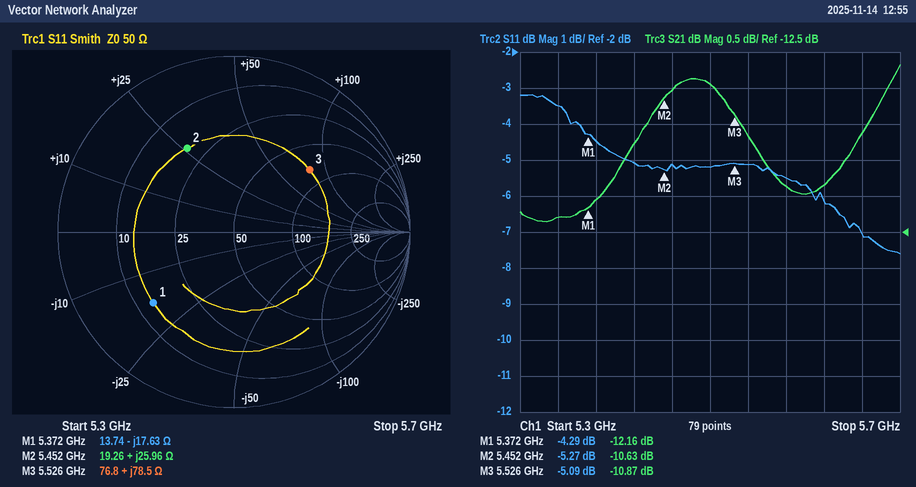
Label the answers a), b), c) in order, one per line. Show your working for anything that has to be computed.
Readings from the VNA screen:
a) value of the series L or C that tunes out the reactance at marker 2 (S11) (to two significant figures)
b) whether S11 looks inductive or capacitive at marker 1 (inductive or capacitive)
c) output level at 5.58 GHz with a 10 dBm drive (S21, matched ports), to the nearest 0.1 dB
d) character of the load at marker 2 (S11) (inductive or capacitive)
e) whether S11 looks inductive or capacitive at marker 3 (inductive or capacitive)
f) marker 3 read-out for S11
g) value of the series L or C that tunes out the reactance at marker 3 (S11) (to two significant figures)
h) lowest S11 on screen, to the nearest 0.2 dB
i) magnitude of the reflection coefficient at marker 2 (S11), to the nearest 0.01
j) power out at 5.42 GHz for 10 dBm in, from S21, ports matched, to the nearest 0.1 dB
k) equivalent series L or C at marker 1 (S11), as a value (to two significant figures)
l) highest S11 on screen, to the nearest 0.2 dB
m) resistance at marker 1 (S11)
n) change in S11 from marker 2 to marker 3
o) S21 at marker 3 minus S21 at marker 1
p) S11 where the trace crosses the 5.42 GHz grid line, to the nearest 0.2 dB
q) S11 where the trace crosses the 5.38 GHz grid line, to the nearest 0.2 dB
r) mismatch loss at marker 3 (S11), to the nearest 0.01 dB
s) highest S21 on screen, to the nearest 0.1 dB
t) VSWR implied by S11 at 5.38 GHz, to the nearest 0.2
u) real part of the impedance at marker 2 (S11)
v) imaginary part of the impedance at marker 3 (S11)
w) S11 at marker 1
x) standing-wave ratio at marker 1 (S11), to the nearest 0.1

a) C = 1/(2π × 5.452 GHz × 25.96 Ω) ≈ 1.1 pF
b) capacitive
c) 10 dBm + (-11.9 dB) = -1.9 dBm
d) inductive
e) inductive
f) -5.09 dB
g) C = 1/(2π × 5.526 GHz × 78.5 Ω) ≈ 367 fF, so 370 fF to two significant figures
h) -7.6 dB
i) 0.54
j) 10 dBm + (-11.3 dB) = -1.3 dBm
k) C = 1/(2π × 5.372 GHz × 17.63 Ω) ≈ 1.7 pF
l) -3.2 dB
m) 13.74 Ω
n) -5.09 − (-5.27) = 0.18 dB
o) -10.87 − (-12.16) = 1.29 dB
p) -5.0 dB
q) -4.4 dB
r) −10 log10(1 − 10^(-5.09/10)) ≈ 1.61 dB
s) -10.2 dB
t) |Γ| = 10^(-4.4/20) = 0.6026; VSWR = (1 + 0.6026)/(1 − 0.6026) ≈ 4.0
u) 19.26 Ω
v) +78.5 Ω
w) -4.29 dB
x) 4.1
